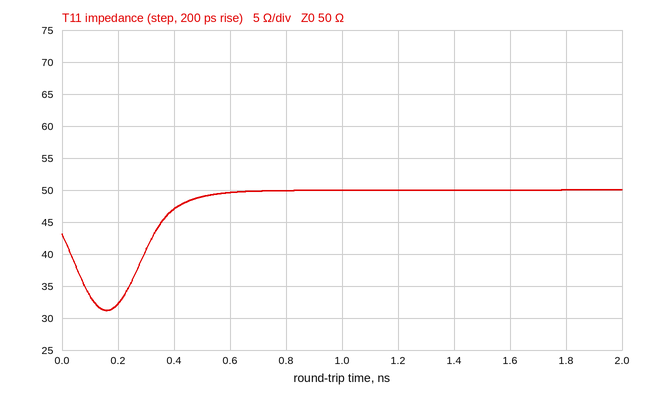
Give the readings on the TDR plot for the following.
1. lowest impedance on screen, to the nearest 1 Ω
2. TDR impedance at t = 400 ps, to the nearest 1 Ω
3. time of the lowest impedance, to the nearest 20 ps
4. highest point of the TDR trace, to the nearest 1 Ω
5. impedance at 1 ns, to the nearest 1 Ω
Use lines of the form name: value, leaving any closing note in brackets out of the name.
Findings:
lowest impedance on screen, to the nearest 1 Ω: 31 Ω
TDR impedance at t = 400 ps, to the nearest 1 Ω: 47 Ω
time of the lowest impedance, to the nearest 20 ps: 160 ps
highest point of the TDR trace, to the nearest 1 Ω: 50 Ω
impedance at 1 ns, to the nearest 1 Ω: 50 Ω
